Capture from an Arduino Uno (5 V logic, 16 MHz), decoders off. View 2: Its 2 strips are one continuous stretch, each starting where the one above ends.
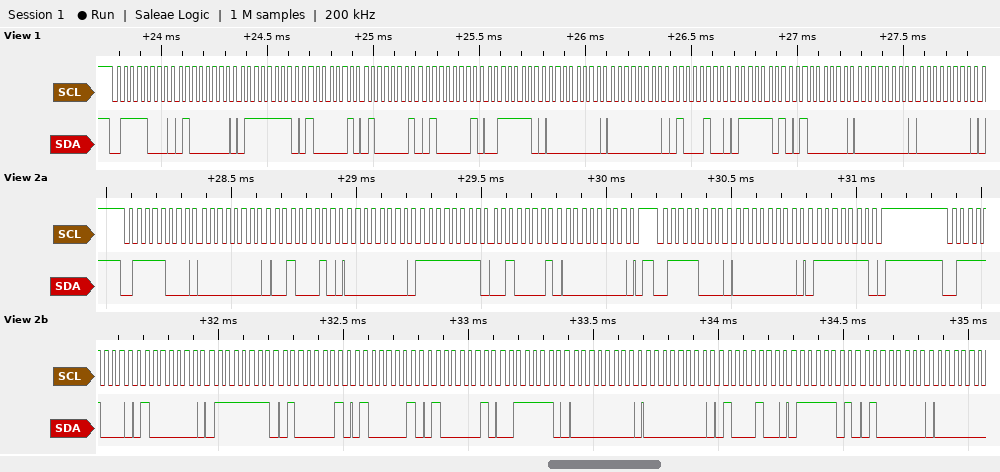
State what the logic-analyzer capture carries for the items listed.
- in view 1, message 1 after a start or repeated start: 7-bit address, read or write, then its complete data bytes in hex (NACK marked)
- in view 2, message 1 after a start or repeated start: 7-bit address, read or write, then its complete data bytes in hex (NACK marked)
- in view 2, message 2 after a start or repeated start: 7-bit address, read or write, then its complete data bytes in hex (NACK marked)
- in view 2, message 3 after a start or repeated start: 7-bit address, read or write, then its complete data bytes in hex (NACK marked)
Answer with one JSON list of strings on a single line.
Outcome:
["0x3C write: 40 7F 41 41 41 3E 00 00 44 7D 40 00 00", "0x3C write: 00 22 00 FF 21 00", "0x3C write: 00 7F", "0x3C write: 40 7F 41 41 41 3E 00 00 44 7D 40"]
